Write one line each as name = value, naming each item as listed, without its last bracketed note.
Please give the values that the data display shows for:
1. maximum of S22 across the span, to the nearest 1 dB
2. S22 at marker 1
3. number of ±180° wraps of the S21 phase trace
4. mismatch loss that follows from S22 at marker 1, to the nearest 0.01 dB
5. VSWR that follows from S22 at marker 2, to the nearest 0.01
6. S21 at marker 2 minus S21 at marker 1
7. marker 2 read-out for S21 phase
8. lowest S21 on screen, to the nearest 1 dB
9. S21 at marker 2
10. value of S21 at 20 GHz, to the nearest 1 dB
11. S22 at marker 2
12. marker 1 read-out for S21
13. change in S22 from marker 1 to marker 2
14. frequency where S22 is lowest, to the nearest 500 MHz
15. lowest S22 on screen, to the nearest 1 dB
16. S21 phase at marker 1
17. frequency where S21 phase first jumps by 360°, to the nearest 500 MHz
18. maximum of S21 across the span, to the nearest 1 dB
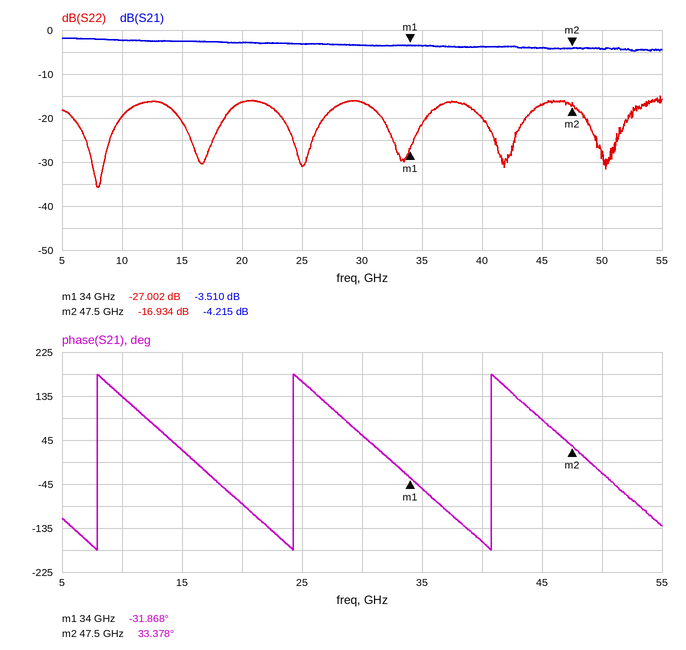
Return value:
maximum of S22 across the span, to the nearest 1 dB = -15 dB
S22 at marker 1 = -27.002 dB
number of ±180° wraps of the S21 phase trace = 3
mismatch loss that follows from S22 at marker 1, to the nearest 0.01 dB = 0.01 dB
VSWR that follows from S22 at marker 2, to the nearest 0.01 = 1.33
S21 at marker 2 minus S21 at marker 1 = -0.705 dB
marker 2 read-out for S21 phase = 33.378°
lowest S21 on screen, to the nearest 1 dB = -5 dB
S21 at marker 2 = -4.215 dB
value of S21 at 20 GHz, to the nearest 1 dB = -3 dB
S22 at marker 2 = -16.934 dB
marker 1 read-out for S21 = -3.510 dB
change in S22 from marker 1 to marker 2 = 10.068 dB
frequency where S22 is lowest, to the nearest 500 MHz = 8.0 GHz
lowest S22 on screen, to the nearest 1 dB = -36 dB
S21 phase at marker 1 = -31.868°
frequency where S21 phase first jumps by 360°, to the nearest 500 MHz = 8.0 GHz
maximum of S21 across the span, to the nearest 1 dB = -2 dB
